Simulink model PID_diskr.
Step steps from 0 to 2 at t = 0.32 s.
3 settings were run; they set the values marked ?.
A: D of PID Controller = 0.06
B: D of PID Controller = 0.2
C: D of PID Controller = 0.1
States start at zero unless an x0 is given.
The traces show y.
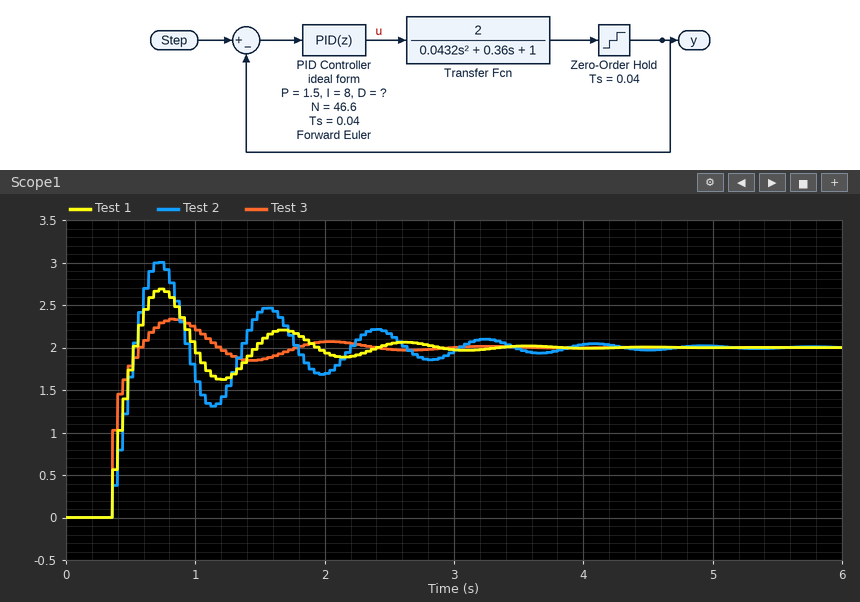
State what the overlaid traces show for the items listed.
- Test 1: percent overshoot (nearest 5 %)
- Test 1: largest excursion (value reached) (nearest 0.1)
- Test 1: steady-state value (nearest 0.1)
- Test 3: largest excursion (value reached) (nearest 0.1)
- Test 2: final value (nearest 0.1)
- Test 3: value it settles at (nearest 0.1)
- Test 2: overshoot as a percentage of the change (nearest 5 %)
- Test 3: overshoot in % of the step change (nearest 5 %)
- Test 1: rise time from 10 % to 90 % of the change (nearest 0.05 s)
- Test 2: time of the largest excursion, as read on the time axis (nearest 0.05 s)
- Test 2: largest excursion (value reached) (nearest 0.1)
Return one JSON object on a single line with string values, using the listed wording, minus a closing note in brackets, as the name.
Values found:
{"Test 1: percent overshoot": "35 %", "Test 1: largest excursion (value reached)": "2.7", "Test 1: steady-state value": "2.0", "Test 3: largest excursion (value reached)": "2.3", "Test 2: final value": "2.0", "Test 3: value it settles at": "2.0", "Test 2: overshoot as a percentage of the change": "50 %", "Test 3: overshoot in % of the step change": "15 %", "Test 1: rise time from 10 % to 90 % of the change": "0.15 s", "Test 2: time of the largest excursion, as read on the time axis": "0.70 s", "Test 2: largest excursion (value reached)": "3.0"}
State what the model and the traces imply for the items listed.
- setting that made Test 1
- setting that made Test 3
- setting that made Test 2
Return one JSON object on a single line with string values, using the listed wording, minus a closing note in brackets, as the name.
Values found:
{"setting that made Test 1": "C", "setting that made Test 3": "B", "setting that made Test 2": "A"}
